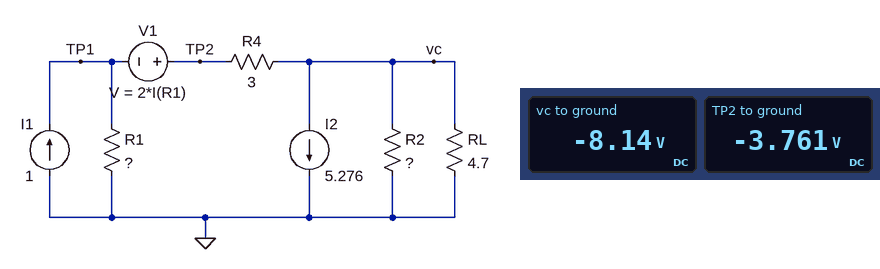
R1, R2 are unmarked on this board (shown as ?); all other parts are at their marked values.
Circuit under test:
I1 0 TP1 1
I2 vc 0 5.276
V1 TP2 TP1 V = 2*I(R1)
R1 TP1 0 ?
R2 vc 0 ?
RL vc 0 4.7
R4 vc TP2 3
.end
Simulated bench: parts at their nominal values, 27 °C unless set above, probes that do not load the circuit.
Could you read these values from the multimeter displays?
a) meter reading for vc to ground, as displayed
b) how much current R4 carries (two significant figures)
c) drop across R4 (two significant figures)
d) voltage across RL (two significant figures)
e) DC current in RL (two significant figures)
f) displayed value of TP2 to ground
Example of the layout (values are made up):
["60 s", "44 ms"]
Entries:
["-8.14 V", "1.5 A", "4.4 V", "8.1 V", "1.7 A", "-3.761 V"]
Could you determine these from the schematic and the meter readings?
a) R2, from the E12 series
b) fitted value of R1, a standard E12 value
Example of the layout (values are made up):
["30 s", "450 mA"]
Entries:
["3.9 Ω", "8.2 Ω"]
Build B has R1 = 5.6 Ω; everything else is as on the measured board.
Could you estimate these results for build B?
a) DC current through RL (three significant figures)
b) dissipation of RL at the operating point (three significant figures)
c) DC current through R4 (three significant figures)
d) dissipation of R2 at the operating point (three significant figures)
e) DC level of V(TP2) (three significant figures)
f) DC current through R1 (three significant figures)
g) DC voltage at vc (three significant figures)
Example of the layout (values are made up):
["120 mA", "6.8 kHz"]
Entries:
["1.68 A", "13.3 W", "1.57 A", "16.0 W", "-3.19 V", "570 mA", "-7.90 V"]
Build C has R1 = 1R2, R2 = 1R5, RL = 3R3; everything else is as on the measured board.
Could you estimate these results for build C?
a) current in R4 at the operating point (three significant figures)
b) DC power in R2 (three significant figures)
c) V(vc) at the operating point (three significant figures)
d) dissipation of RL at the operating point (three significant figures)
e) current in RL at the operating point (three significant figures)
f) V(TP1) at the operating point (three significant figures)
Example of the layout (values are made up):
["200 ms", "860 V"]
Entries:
["1.27 A", "11.4 W", "-4.13 V", "5.17 W", "1.25 A", "-323 mV"]
